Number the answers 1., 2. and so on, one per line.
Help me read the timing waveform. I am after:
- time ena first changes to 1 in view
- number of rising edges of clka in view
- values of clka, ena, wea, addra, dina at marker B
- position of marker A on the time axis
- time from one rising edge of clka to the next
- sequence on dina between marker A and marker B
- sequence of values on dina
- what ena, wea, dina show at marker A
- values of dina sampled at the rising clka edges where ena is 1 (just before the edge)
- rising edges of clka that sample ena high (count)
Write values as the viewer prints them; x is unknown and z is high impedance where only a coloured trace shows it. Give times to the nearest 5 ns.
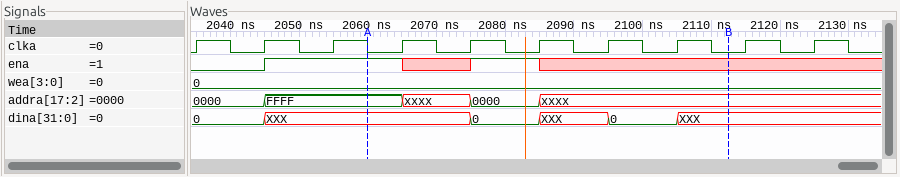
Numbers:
1. 2045 ns
2. 10
3. clka=0, ena=x, wea=0, addra=xxxx, dina=XXX
4. 2060 ns
5. 10 ns
6. XXX, 0, XXX, 0, XXX
7. 0, XXX, 0, XXX, 0, XXX
8. ena=1, wea=0, dina=XXX
9. XXX, XXX, 0
10. 3
